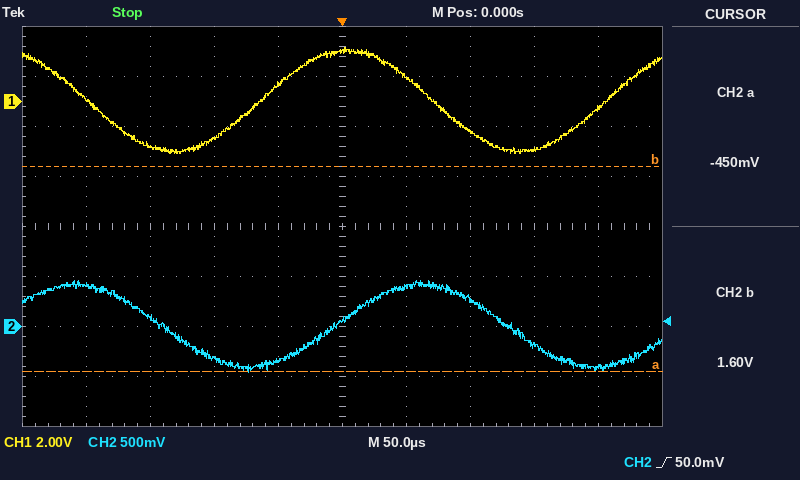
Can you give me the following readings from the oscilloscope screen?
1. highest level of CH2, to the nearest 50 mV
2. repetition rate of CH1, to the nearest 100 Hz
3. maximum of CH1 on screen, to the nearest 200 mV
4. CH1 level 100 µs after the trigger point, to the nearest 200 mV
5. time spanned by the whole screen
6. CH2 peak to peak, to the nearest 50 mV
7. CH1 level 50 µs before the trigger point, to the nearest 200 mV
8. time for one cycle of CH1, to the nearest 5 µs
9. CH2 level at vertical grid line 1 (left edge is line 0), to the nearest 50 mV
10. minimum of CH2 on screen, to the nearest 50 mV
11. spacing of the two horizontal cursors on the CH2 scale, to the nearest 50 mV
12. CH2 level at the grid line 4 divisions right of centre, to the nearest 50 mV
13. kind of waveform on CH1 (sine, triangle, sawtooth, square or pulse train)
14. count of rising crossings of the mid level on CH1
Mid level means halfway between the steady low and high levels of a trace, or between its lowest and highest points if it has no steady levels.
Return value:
450 mV
3.7 kHz
2.2 V
-1.2 V
500 µs
900 mV
600 mV
270 µs
400 mV
-450 mV
2.05 V
-400 mV
sine
2
